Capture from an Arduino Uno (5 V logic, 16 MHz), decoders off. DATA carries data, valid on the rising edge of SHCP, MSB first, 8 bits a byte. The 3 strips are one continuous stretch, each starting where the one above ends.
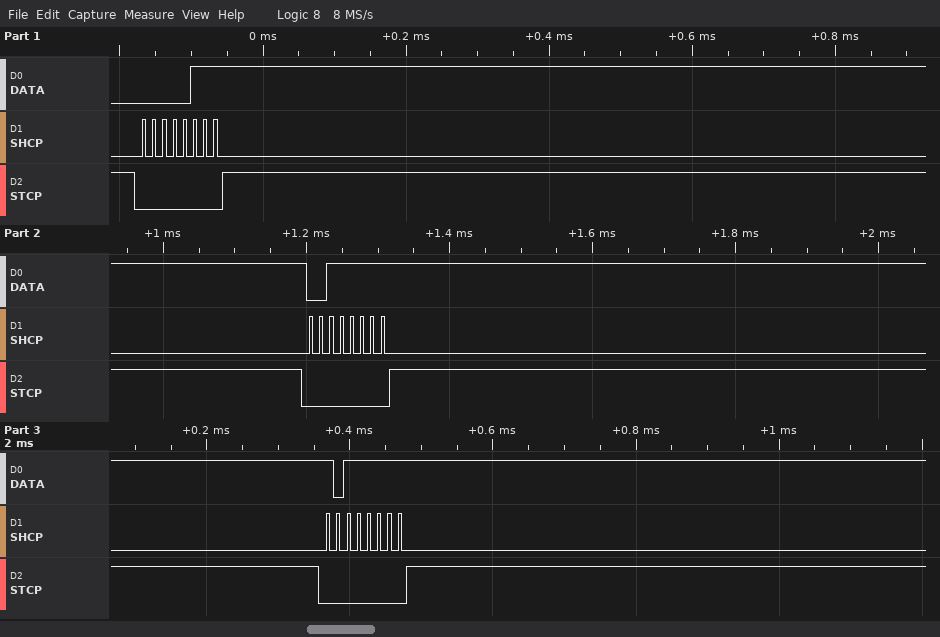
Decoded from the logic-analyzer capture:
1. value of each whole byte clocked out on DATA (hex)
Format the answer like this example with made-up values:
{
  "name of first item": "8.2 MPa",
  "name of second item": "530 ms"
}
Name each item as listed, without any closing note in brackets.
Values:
{
  "value of each whole byte clocked out on DATA": "0x07 0x3F 0xBF"
}
